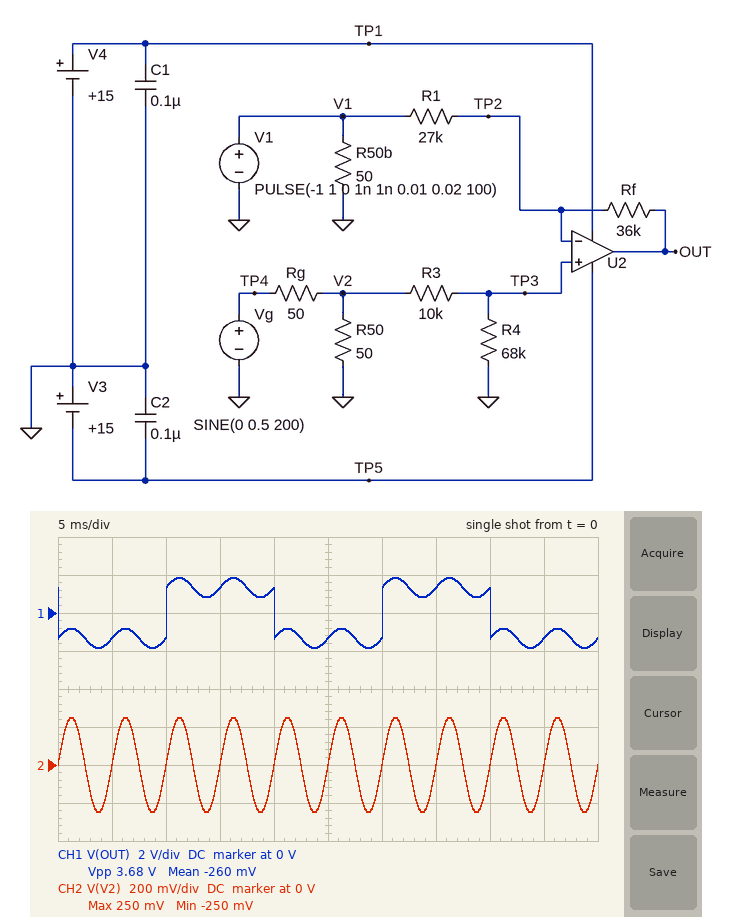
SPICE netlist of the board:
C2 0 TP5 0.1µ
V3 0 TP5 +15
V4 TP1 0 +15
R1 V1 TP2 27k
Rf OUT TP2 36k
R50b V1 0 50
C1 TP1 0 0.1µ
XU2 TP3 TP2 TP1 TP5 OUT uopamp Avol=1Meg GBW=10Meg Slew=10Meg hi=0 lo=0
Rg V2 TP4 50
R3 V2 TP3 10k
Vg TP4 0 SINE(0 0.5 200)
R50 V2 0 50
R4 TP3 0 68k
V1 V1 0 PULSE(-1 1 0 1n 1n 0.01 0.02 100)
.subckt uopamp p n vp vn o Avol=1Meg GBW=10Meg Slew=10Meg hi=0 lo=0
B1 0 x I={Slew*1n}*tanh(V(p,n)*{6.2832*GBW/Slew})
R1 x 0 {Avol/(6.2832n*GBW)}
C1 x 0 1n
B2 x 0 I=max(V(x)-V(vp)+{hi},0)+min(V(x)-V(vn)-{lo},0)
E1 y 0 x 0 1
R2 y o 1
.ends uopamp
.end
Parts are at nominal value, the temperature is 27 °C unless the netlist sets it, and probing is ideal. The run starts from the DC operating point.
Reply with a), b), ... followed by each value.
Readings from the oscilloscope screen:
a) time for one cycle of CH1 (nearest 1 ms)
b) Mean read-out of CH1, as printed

a) 20 ms
b) -260 mV
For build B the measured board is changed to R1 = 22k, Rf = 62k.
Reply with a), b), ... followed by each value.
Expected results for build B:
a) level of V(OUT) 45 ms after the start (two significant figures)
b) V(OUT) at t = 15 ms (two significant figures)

a) -2.8 V
b) 2.8 V
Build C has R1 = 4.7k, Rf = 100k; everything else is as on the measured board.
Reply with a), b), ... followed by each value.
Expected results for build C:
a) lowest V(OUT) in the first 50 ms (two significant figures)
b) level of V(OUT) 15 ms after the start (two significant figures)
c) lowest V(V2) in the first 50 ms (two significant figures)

a) -15 V
b) 15 V
c) -250 mV
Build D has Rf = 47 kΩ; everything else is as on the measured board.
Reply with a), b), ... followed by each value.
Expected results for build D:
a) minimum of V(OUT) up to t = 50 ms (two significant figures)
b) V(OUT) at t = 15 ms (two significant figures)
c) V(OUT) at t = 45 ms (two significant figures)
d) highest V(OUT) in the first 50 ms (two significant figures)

a) -2.3 V
b) 1.7 V
c) -1.7 V
d) 2.3 V
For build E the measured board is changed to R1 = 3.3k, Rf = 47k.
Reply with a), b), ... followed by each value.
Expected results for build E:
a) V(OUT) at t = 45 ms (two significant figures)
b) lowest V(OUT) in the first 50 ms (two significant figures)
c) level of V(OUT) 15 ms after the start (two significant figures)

a) -14 V
b) -15 V
c) 14 V
